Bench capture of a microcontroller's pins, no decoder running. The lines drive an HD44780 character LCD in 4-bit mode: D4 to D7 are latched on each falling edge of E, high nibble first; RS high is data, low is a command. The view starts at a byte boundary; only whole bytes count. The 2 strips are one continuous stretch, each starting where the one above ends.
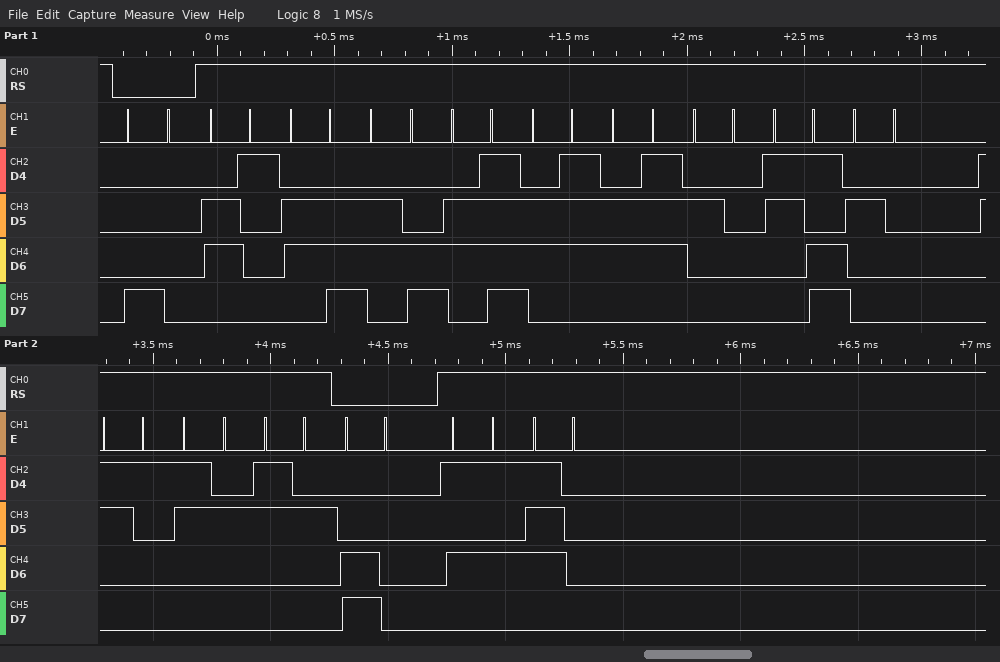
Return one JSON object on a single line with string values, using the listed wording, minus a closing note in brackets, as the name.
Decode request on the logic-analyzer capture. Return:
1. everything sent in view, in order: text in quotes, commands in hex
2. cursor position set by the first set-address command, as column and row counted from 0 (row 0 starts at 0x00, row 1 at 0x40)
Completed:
{"everything sent in view, in order: text in quotes, commands in hex": "0x80 \"anlogg = 122\" 0xC0 \"Up\"", "cursor position set by the first set-address command, as column and row counted from 0": "column 0, row 0"}
